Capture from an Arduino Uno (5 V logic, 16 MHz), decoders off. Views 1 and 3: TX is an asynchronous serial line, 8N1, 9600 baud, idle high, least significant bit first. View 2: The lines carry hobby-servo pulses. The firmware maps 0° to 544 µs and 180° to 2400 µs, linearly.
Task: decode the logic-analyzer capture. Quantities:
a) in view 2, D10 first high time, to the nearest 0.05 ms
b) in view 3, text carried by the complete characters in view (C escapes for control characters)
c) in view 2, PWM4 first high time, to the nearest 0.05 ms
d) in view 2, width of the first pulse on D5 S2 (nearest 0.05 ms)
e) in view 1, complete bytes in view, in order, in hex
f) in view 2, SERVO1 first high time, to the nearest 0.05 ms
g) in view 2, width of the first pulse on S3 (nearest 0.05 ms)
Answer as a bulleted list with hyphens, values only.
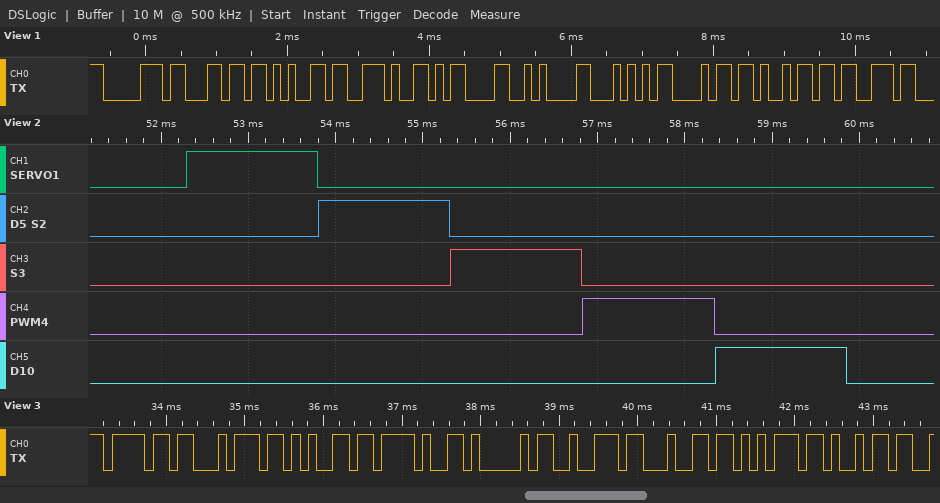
- 1.50 ms
- "ote/Ardui"
- 1.50 ms
- 1.50 ms
- 0x70 0x6C 0x65 0x2E 0x0D 0x0A 0x54 0x68 0x69 0x73
- 1.50 ms
- 1.50 ms
